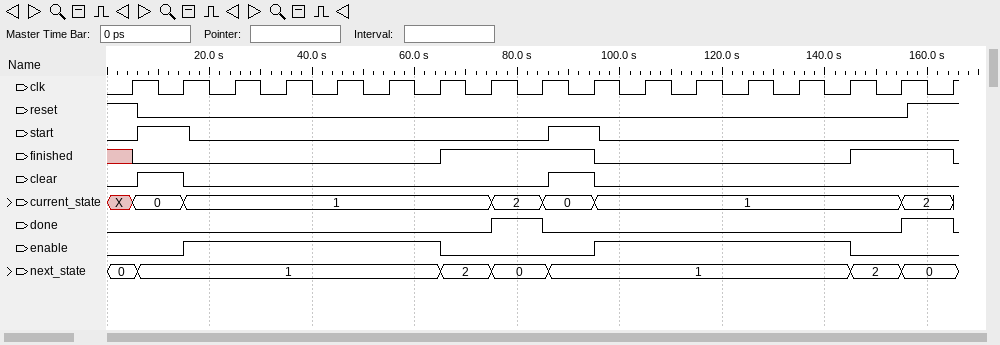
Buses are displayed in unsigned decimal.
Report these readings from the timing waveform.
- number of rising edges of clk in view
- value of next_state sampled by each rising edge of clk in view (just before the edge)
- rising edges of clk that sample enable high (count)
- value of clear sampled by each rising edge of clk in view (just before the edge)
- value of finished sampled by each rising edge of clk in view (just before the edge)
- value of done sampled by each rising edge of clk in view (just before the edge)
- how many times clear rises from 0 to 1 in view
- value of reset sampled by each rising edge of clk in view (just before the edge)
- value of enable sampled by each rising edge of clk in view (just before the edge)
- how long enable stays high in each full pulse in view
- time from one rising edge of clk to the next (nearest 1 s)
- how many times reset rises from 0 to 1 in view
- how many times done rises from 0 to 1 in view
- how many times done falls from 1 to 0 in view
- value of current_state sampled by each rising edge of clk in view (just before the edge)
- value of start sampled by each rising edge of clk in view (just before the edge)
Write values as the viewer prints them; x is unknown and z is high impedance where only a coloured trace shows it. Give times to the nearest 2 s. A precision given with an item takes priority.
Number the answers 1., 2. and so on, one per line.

1. 17
2. 0, 1, 1, 1, 1, 1, 1, 2, 0, 1, 1, 1, 1, 1, 1, 2, 0
3. 10
4. 0 1 0 0 0 0 0 0 0 1 0 0 0 0 0 0 0
5. x 0 0 0 0 0 0 1 1 1 0 0 0 0 0 1 1
6. 0 0 0 0 0 0 0 0 1 0 0 0 0 0 0 0 1
7. 2
8. 1 0 0 0 0 0 0 0 0 0 0 0 0 0 0 0 1
9. 0 0 1 1 1 1 1 0 0 0 1 1 1 1 1 0 0
10. 50 s, 50 s
11. 10 s
12. 1
13. 2
14. 2
15. X, 0, 1, 1, 1, 1, 1, 1, 2, 0, 1, 1, 1, 1, 1, 1, 2
16. 0 1 0 0 0 0 0 0 0 1 0 0 0 0 0 0 0
